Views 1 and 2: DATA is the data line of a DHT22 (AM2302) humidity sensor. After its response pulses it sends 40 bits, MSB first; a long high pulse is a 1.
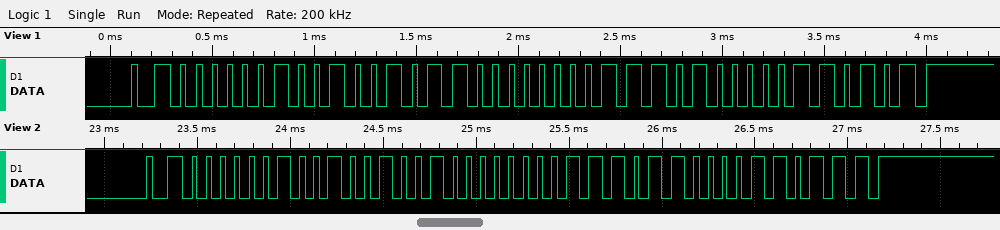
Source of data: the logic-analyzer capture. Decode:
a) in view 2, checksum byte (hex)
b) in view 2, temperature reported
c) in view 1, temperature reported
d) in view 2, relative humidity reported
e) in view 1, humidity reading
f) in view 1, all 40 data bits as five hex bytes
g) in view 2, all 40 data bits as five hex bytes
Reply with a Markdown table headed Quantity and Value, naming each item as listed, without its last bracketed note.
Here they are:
| Quantity | Value |
|---|---|
| in view 2, checksum byte | 0x37 |
| in view 2, temperature reported | 23.6 °C |
| in view 1, temperature reported | 23.2 °C |
| in view 2, relative humidity reported | 58.5 % |
| in view 1, humidity reading | 58.7 % |
| in view 1, all 40 data bits as five hex bytes | 02 4B 00 E8 35 |
| in view 2, all 40 data bits as five hex bytes | 02 49 00 EC 37 |
